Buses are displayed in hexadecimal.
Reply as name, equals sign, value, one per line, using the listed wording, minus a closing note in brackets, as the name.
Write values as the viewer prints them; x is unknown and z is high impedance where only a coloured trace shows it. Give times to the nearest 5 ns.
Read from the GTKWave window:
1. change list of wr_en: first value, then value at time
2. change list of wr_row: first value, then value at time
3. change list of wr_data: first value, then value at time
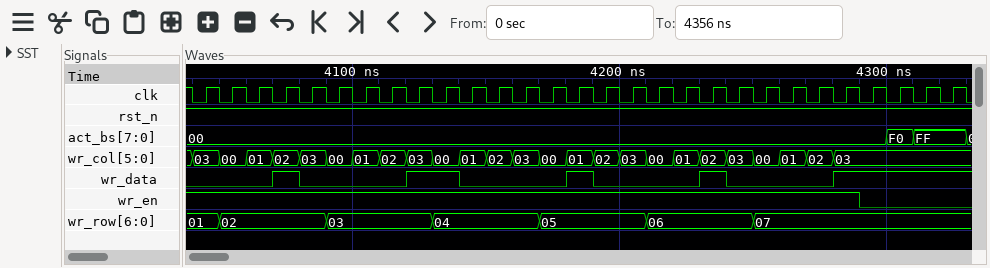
change list of wr_en: first value, then value at time = 1, 0 at 4290 ns
change list of wr_row: first value, then value at time = 01, 02 at 4050 ns, 03 at 4090 ns, 04 at 4130 ns, 05 at 4170 ns, 06 at 4210 ns, 07 at 4250 ns
change list of wr_data: first value, then value at time = 0, 1 at 4070 ns, 0 at 4080 ns, 1 at 4120 ns, 0 at 4140 ns, 1 at 4180 ns, 0 at 4190 ns, 1 at 4230 ns, 0 at 4240 ns, 1 at 4280 ns
